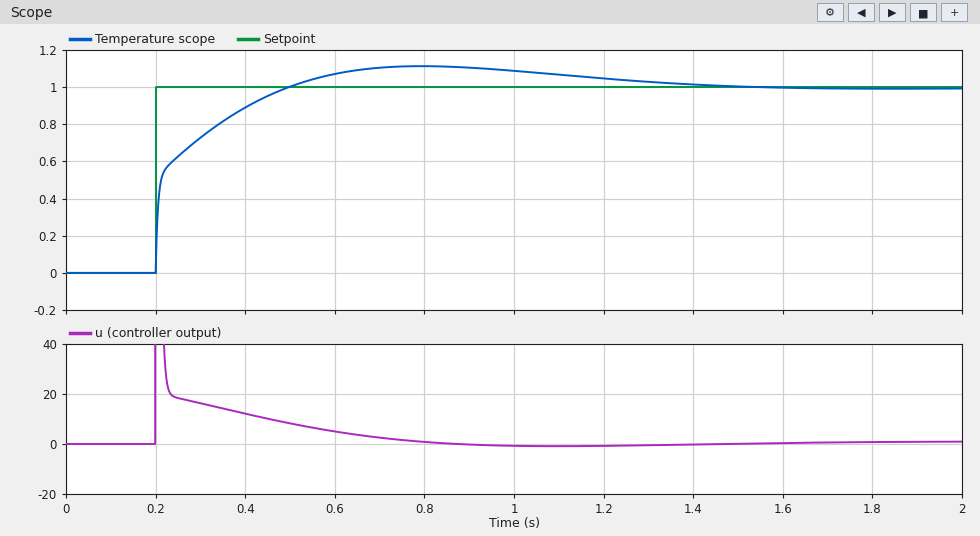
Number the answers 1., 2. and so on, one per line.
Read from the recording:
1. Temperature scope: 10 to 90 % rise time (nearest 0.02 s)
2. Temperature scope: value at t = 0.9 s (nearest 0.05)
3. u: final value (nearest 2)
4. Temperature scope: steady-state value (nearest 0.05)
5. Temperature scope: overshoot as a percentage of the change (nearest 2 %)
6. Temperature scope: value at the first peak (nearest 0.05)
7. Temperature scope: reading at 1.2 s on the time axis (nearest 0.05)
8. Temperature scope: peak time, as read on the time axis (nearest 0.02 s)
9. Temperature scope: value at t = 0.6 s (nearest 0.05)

1. 0.20 s
2. 1.10
3. 0
4. 1.00
5. 12 %
6. 1.10
7. 1.05
8. 0.80 s
9. 1.05
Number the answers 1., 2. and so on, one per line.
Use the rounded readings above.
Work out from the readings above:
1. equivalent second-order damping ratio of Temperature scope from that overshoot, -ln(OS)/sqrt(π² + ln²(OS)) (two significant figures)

1. 0.56
